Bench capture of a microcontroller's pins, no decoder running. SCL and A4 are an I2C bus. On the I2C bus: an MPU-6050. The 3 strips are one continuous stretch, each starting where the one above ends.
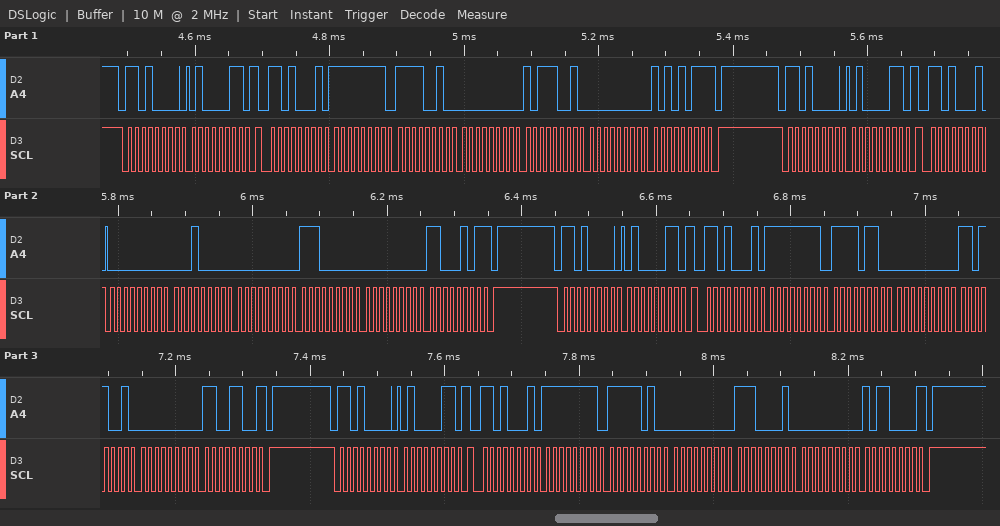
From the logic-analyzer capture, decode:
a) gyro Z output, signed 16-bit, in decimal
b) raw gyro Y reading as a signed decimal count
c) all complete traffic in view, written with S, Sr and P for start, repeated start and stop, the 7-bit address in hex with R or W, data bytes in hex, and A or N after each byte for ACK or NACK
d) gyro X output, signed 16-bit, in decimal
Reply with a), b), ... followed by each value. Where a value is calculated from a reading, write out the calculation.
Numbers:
a) 0x00AB = 171
b) 0x00B9 = 185
c) S 68W A 43 A Sr 68R A FF A F2 A 00 A B9 A 00 A AB N P S 68W A 43 A Sr 68R A 00 A 10 A 00 A E0 A 00 A C5 N P S 68W A 43 A Sr 68R A FF A F6 A 00 A D9 A 00 A CC N P S 68W A 43 A Sr 68R A FF A FA A 00 A E1 A 00 A B0 N P
d) 0xFFF2 = -14
